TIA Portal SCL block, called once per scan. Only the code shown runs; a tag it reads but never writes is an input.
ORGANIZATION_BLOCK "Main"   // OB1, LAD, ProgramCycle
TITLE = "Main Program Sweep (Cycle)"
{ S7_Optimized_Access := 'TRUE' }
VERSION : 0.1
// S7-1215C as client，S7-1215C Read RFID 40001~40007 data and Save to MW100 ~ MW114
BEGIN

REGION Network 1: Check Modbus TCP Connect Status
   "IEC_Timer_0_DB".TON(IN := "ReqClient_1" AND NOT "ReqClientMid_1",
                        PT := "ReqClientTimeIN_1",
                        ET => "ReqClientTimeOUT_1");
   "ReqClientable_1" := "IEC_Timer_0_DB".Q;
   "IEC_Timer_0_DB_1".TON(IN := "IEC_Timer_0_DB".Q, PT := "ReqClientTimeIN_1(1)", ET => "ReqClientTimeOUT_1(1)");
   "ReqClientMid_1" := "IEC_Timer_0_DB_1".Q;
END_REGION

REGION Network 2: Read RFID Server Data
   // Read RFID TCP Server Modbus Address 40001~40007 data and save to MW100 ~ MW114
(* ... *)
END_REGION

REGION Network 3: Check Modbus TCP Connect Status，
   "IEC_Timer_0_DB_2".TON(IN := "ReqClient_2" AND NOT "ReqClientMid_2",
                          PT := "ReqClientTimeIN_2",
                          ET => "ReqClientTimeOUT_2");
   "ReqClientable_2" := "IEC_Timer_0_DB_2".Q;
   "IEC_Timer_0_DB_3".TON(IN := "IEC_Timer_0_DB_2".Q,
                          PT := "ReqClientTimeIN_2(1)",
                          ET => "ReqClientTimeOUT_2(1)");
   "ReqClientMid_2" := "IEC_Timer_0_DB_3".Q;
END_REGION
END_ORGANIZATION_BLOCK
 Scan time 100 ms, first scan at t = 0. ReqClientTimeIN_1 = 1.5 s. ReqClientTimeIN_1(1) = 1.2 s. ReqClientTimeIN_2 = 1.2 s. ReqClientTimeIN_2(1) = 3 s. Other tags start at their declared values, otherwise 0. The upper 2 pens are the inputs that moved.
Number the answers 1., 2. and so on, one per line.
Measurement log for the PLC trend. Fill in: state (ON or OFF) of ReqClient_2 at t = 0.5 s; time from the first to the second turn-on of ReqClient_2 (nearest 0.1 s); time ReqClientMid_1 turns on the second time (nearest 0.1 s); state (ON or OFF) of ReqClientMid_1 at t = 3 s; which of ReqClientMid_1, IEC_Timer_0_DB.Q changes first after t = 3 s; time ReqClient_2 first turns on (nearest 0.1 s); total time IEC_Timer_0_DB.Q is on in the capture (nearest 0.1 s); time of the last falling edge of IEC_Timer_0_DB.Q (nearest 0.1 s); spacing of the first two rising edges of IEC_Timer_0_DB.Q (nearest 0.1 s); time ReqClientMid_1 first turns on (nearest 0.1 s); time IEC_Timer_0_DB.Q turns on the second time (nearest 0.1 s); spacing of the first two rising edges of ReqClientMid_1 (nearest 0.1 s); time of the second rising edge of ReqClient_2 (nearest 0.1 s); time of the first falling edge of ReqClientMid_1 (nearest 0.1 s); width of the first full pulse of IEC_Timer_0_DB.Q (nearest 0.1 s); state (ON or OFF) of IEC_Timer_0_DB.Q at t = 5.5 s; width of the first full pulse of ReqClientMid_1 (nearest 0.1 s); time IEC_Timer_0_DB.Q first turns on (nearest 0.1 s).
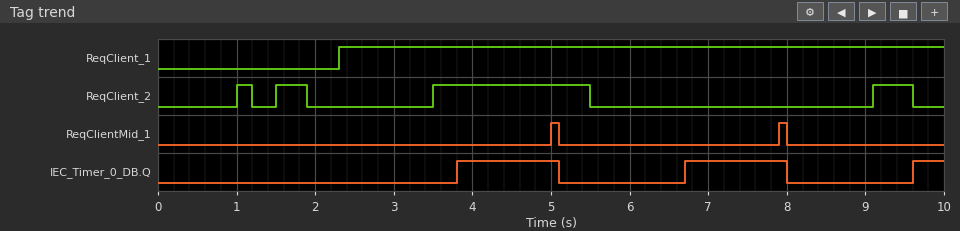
1. OFF
2. 0.5 s
3. 7.9 s
4. OFF
5. IEC_Timer_0_DB.Q
6. 1.0 s
7. 3.0 s
8. 8.0 s
9. 2.9 s
10. 5.0 s
11. 6.7 s
12. 2.9 s
13. 1.5 s
14. 5.1 s
15. 1.3 s
16. OFF
17. 0.1 s
18. 3.8 s
